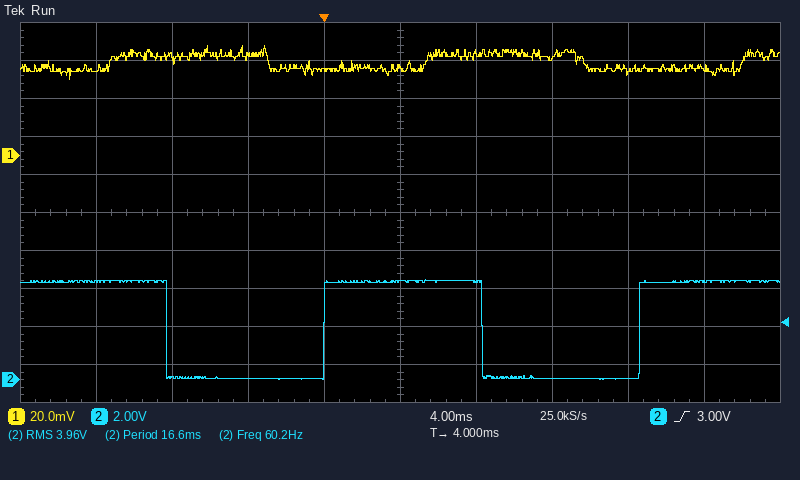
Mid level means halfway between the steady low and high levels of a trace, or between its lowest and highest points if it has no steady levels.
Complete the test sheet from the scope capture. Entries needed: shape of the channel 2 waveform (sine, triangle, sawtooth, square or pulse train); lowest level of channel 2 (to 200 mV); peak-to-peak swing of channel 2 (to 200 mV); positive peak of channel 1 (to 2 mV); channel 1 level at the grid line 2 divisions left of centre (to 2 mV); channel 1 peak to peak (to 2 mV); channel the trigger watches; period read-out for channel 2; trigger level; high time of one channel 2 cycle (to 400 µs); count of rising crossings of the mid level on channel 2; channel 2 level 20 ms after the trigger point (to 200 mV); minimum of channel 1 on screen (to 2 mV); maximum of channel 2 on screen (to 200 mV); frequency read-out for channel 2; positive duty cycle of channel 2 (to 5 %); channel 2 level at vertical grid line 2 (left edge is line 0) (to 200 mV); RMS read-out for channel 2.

square
0.0 V
5.2 V
58 mV
52 mV
18 mV
channel 2
16.6 ms
3.00 V
8.4 ms
2
5.2 V
40 mV
5.2 V
60.2 Hz
50 %
200 mV
3.96 V
